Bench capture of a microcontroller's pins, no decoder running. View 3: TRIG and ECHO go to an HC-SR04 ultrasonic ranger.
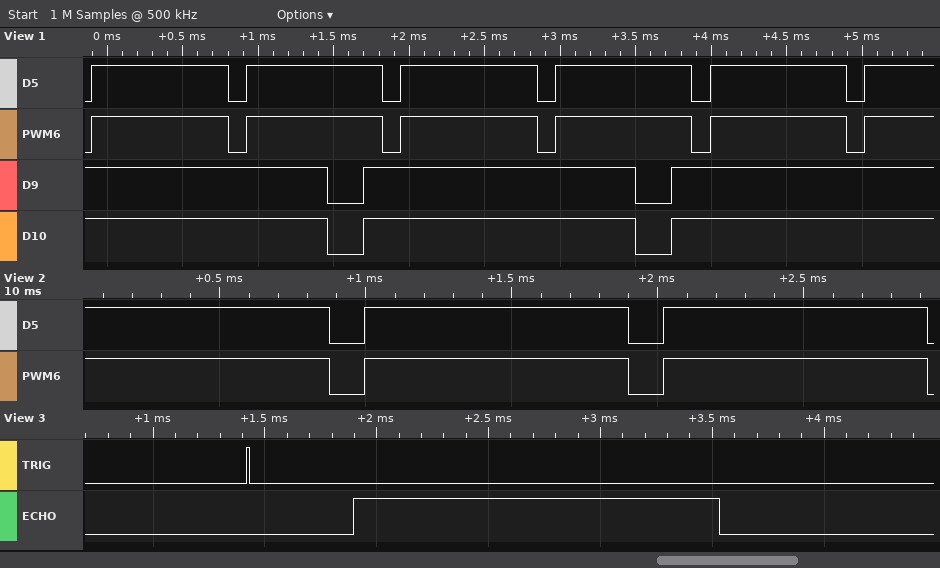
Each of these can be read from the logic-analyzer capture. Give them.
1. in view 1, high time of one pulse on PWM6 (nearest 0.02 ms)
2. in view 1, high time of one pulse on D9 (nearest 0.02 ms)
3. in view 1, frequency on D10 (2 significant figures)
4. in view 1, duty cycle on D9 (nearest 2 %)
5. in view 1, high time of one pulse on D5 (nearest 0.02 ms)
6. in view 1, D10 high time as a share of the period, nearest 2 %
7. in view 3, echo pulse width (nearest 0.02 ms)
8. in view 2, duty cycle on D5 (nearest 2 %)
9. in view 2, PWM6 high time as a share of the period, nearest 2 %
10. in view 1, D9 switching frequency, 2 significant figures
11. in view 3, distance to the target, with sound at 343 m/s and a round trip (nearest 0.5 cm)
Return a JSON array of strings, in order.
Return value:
["0.90 ms", "1.80 ms", "490 Hz", "88 %", "0.90 ms", "88 %", "1.64 ms", "88 %", "88 %", "490 Hz", "28 cm"]
